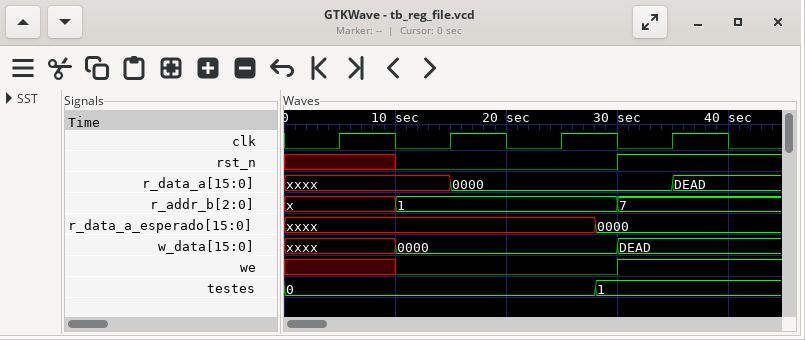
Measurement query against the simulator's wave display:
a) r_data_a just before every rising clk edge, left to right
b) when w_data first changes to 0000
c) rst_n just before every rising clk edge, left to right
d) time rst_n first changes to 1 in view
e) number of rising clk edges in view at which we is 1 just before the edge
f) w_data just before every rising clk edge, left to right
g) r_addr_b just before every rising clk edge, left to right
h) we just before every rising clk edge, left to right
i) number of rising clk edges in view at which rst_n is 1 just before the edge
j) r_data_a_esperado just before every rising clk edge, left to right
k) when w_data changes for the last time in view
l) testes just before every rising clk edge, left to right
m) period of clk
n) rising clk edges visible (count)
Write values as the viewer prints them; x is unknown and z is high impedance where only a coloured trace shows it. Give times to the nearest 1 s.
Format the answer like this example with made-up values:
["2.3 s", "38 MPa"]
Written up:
["xxxx, xxxx, 0000, 0000", "10 s", "x 0 0 1", "30 s", "1", "xxxx, 0000, 0000, DEAD", "x, 1, 1, 7", "x 0 0 1", "1", "xxxx, xxxx, xxxx, 0000", "30 s", "0, 0, 0, 1", "10 s", "4"]
